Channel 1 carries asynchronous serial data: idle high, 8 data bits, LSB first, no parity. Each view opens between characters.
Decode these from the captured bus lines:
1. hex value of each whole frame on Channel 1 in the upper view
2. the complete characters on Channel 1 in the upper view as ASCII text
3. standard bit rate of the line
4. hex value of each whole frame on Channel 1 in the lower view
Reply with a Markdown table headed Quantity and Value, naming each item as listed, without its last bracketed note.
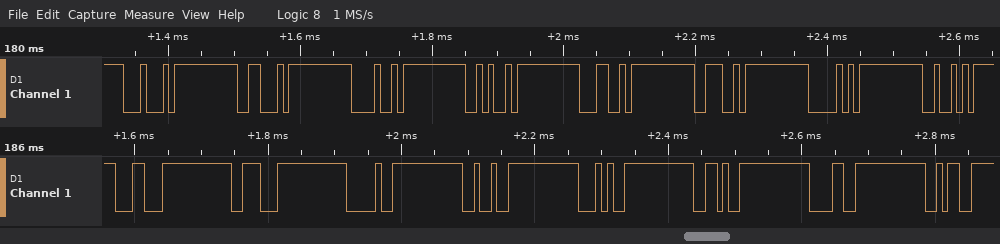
| Quantity | Value |
|---|---|
| hex value of each whole frame on Channel 1 in the upper view | 44, 46, 48, 4A, 4C, 4E, 50, 52 |
| the complete characters on Channel 1 in the upper view as ASCII text | "DFHJLNPR" |
| standard bit rate of the line | 115200 baud |
| hex value of each whole frame on Channel 1 in the lower view | 8C, 8E, 90, 92, 94, 96, 98, 9A |
